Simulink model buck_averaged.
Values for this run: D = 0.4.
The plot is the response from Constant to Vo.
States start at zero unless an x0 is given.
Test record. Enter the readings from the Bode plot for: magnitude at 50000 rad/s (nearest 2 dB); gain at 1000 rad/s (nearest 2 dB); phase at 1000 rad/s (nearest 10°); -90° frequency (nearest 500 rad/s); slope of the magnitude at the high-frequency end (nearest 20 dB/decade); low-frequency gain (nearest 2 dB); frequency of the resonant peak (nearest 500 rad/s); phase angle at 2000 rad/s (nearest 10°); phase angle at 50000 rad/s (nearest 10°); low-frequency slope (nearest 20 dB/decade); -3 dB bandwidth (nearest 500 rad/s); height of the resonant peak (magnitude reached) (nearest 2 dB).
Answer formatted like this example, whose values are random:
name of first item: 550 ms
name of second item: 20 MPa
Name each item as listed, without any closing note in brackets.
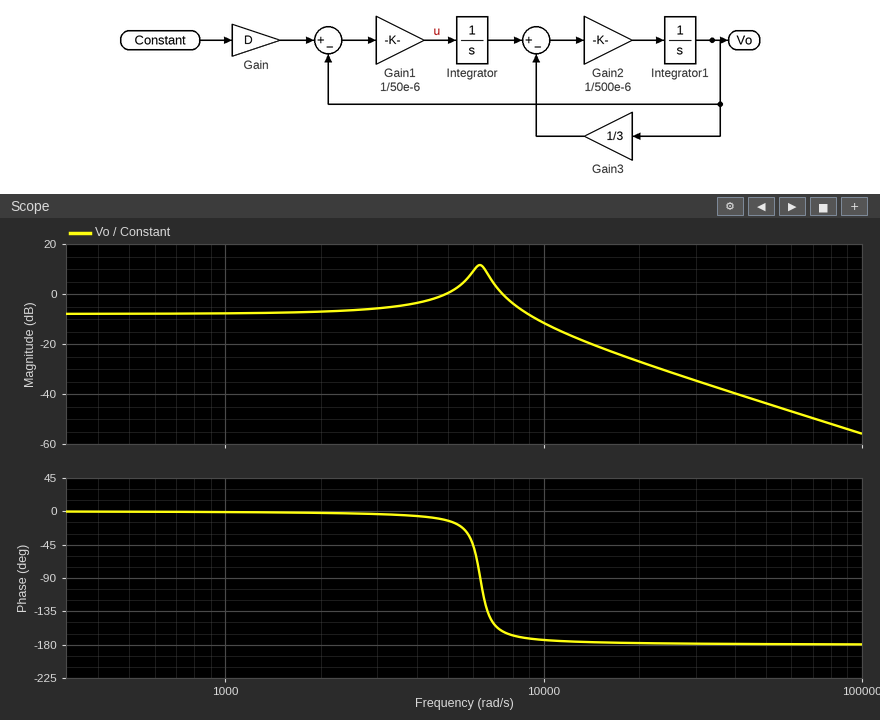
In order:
magnitude at 50000 rad/s: -44 dB
gain at 1000 rad/s: -8 dB
phase at 1000 rad/s: 0°
-90° frequency: 6500 rad/s
slope of the magnitude at the high-frequency end: -40 dB/decade
low-frequency gain: -8 dB
frequency of the resonant peak: 6500 rad/s
phase angle at 2000 rad/s: 0°
phase angle at 50000 rad/s: -180°
low-frequency slope: 0 dB/decade
-3 dB bandwidth: 10000 rad/s
height of the resonant peak (magnitude reached): 12 dB
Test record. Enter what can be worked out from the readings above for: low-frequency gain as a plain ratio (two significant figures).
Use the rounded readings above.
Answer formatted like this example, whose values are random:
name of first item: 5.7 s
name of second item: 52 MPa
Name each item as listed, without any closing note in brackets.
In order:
low-frequency gain as a plain ratio: 0.40
